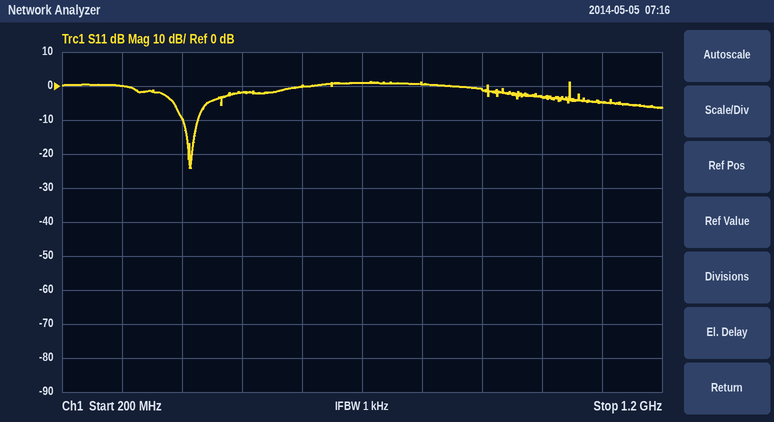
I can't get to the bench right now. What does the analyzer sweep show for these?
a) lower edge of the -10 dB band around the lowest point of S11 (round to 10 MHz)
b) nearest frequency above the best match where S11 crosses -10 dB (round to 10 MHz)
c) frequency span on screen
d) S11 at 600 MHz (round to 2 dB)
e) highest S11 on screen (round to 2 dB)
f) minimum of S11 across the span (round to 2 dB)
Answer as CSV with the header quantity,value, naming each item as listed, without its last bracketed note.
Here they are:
quantity,value
lower edge of the -10 dB band around the lowest point of S11,400 MHz
nearest frequency above the best match where S11 crosses -10 dB,430 MHz
frequency span on screen,1 GHz
S11 at 600 MHz,0 dB
highest S11 on screen,2 dB
minimum of S11 across the span,-24 dB
